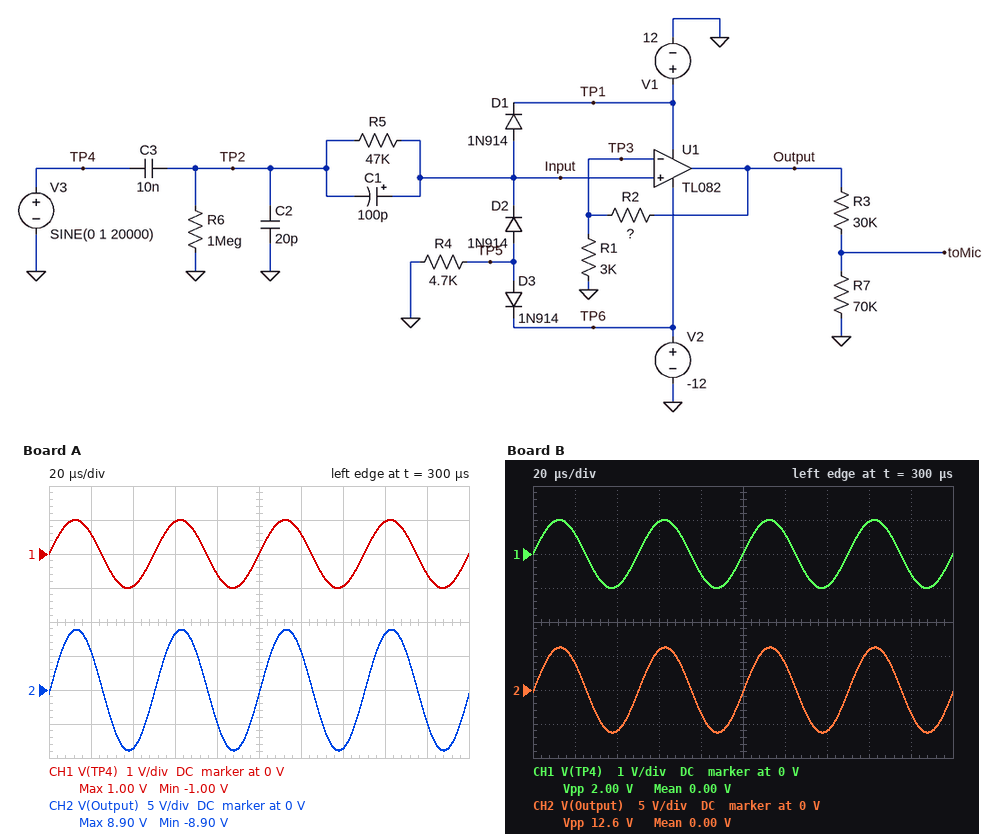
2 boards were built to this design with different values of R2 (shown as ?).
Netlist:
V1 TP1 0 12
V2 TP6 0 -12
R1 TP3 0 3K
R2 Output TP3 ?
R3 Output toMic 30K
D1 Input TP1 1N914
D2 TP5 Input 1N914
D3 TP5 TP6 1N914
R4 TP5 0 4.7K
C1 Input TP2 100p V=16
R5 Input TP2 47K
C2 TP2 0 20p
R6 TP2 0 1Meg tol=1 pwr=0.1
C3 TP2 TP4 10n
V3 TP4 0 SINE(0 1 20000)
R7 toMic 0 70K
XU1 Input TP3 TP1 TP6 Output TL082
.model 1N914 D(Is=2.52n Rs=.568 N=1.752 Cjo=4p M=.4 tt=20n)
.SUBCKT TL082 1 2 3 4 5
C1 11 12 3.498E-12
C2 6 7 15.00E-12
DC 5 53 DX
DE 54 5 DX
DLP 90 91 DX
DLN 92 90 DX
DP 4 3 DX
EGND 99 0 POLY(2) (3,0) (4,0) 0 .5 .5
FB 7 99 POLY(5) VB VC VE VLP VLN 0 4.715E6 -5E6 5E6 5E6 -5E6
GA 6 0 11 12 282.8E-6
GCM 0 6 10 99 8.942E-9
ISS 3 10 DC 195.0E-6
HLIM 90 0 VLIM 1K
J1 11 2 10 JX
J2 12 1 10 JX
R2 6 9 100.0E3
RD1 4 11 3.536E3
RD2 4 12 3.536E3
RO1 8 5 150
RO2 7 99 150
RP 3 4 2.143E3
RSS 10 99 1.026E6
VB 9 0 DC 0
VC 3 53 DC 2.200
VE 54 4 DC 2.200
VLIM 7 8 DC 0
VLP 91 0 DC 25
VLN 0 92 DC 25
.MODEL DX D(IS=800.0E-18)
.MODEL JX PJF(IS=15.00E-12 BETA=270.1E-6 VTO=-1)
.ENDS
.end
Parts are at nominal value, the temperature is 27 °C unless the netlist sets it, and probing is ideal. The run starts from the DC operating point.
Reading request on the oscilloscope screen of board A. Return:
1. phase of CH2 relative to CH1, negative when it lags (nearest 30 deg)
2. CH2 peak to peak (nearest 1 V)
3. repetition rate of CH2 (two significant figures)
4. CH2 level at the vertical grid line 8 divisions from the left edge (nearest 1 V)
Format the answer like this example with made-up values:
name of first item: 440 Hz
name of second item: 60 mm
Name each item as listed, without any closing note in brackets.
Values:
phase of CH2 relative to CH1, negative when it lags: 0 deg
CH2 peak to peak: 18 V
repetition rate of CH2: 20 kHz
CH2 level at the vertical grid line 8 divisions from the left edge: 8 V
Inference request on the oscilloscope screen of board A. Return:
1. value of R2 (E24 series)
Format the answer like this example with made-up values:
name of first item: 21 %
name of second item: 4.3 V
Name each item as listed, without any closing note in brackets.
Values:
value of R2: 24 kΩ
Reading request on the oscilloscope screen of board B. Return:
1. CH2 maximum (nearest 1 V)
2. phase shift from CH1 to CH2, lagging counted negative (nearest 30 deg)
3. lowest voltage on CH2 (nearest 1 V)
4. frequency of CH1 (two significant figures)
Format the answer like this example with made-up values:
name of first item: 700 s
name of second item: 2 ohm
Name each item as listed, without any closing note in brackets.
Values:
CH2 maximum: 6 V
phase shift from CH1 to CH2, lagging counted negative: 0 deg
lowest voltage on CH2: -6 V
frequency of CH1: 20 kHz
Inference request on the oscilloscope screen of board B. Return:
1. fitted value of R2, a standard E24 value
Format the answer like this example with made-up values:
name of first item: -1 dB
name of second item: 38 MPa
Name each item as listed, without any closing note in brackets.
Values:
fitted value of R2, a standard E24 value: 16 kΩ
